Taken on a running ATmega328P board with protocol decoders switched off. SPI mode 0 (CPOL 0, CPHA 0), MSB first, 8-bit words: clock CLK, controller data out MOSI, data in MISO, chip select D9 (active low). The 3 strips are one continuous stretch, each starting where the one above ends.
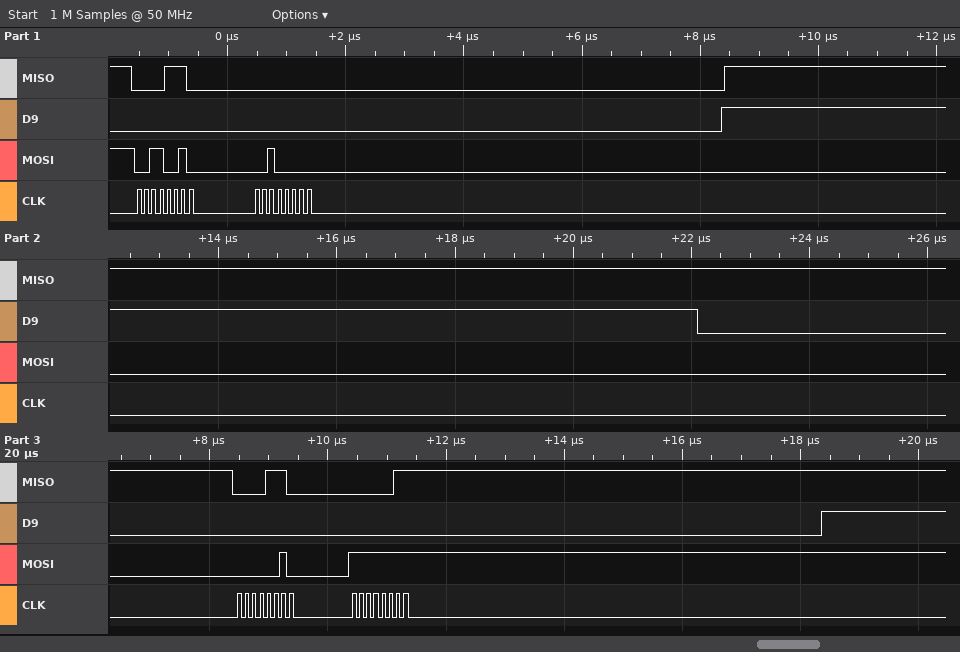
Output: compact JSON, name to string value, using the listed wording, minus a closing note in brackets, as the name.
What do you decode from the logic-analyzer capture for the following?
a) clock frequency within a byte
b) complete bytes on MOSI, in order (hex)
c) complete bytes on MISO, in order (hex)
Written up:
{"clock frequency within a byte": "8 MHz", "complete bytes on MOSI, in order": "32 20 02 FF", "complete bytes on MISO, in order": "0E 00 0E 03"}
